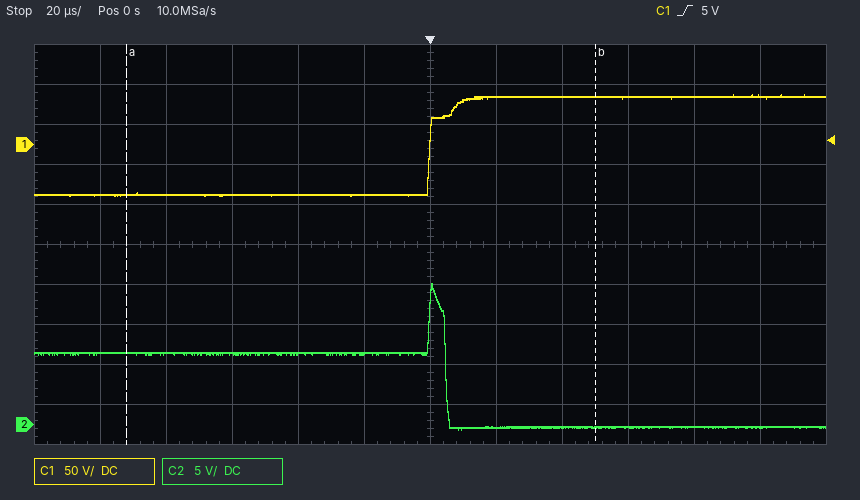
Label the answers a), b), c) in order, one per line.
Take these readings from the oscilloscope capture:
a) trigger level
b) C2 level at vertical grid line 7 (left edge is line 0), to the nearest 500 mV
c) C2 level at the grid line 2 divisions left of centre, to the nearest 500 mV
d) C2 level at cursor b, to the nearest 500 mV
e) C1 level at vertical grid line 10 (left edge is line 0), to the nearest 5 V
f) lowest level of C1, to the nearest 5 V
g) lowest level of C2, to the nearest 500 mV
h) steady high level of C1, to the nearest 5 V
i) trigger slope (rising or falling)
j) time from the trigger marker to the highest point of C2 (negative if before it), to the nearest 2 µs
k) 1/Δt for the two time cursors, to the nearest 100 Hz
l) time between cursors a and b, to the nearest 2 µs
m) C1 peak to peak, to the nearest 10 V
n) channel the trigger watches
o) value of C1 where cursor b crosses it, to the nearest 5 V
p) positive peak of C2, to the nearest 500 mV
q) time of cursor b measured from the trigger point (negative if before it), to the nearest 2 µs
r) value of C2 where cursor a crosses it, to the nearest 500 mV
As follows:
a) 5 V
b) -500 mV
c) 9.0 V
d) -500 mV
e) 60 V
f) -65 V
g) -500 mV
h) 60 V
i) rising
j) 0 µs
k) 7.0 kHz
l) 142 µs
m) 130 V
n) C1
o) 60 V
p) 17.5 V
q) +50 µs
r) 9.0 V
